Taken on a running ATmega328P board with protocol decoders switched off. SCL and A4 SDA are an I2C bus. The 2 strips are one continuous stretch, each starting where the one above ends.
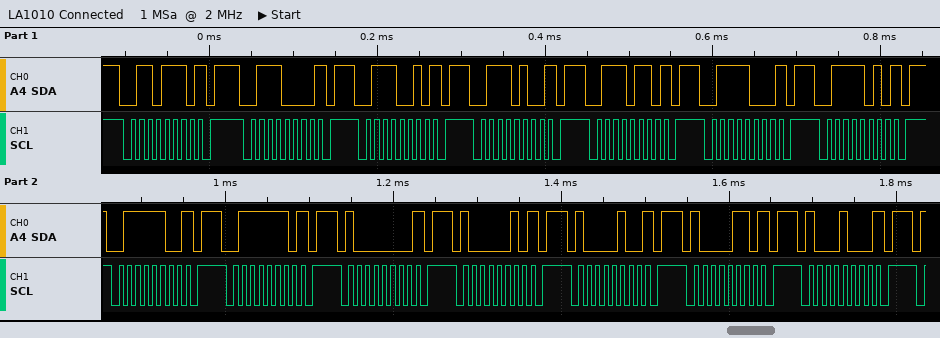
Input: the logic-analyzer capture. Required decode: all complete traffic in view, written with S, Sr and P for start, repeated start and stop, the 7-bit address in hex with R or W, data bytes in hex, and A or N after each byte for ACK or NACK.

S 37W N P S 38W N P S 39W N P S 3AW N P S 3BW N P S 3CW N P S 3DW N P S 3EW N P S 3FW N P S 40W N P S 41W N P S 42W N P S 43W N P S 44W N P
